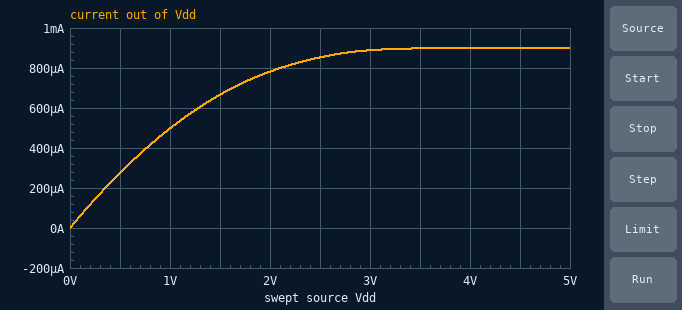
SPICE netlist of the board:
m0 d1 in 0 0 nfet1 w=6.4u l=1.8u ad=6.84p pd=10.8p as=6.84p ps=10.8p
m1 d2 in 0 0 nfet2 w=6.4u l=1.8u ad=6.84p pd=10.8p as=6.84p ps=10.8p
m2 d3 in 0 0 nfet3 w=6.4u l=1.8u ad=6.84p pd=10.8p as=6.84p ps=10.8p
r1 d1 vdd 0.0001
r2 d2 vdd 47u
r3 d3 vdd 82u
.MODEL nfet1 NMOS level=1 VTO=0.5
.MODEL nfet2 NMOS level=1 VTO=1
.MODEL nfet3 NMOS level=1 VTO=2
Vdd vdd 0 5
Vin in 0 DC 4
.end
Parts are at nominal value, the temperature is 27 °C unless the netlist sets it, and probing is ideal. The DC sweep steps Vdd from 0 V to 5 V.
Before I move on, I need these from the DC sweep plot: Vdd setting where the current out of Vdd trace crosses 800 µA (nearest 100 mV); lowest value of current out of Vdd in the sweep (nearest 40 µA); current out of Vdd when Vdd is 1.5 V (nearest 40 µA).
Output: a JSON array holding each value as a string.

["2.1 V", "0 A", "680 µA"]
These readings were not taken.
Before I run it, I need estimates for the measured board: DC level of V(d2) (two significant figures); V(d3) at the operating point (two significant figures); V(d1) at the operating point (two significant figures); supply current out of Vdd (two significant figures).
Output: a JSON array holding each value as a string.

["5.0 V", "5.0 V", "5.0 V", "900 µA"]
